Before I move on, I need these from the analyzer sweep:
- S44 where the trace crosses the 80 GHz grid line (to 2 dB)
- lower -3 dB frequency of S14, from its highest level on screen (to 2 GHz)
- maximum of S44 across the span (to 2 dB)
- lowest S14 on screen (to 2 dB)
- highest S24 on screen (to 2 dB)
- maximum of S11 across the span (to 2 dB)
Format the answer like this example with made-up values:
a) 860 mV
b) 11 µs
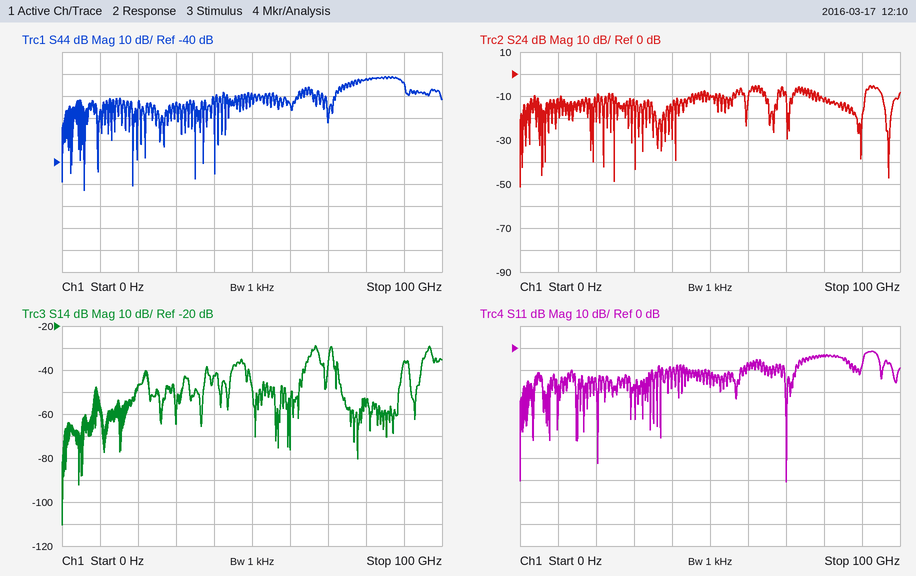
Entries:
a) -2 dB
b) 66 GHz
c) -2 dB
d) -110 dB
e) -6 dB
f) -2 dB
